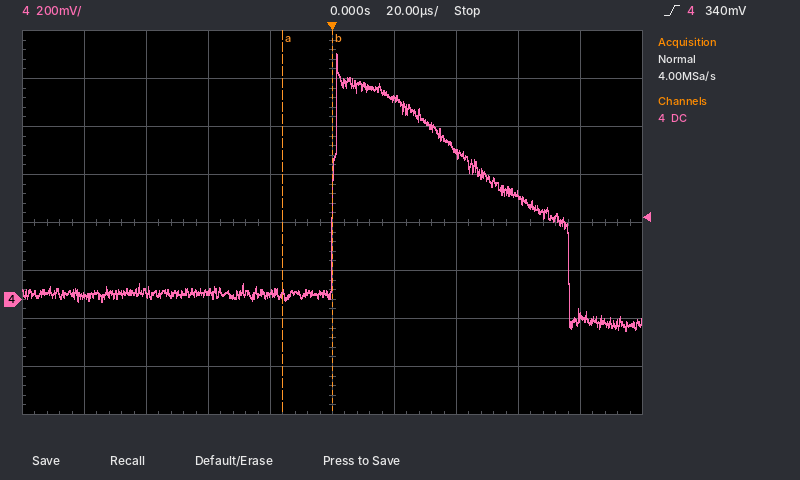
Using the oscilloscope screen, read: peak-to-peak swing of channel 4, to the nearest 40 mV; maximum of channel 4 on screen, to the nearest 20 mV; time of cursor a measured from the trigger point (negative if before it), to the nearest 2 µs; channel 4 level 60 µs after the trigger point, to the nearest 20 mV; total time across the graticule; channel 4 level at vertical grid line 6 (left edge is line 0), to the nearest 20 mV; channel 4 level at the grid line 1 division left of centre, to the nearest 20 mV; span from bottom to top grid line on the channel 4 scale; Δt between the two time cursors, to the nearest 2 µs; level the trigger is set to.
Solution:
1.16 V
1.02 V
-16 µs
440 mV
200 µs
840 mV
20 mV
1.6 V
16 µs
340 mV
